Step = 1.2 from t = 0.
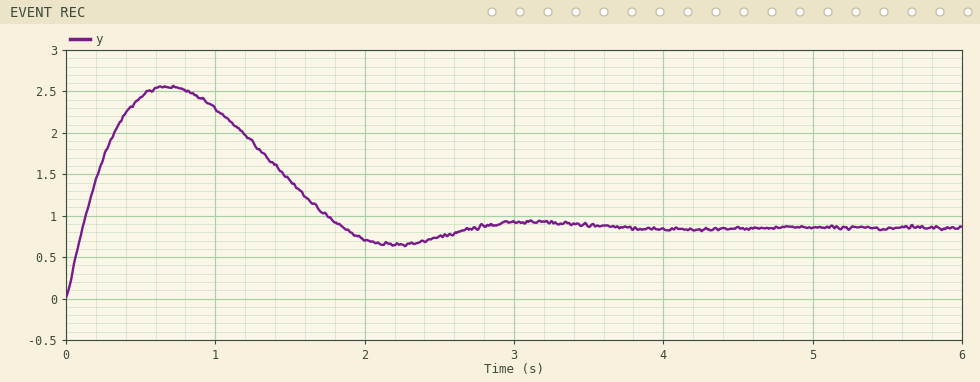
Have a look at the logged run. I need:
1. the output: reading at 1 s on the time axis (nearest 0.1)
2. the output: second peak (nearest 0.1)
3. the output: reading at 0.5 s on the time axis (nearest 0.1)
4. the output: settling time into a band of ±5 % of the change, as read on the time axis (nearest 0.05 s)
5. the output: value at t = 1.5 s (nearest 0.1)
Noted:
2.3
0.9
2.4
3.45 s
1.4
